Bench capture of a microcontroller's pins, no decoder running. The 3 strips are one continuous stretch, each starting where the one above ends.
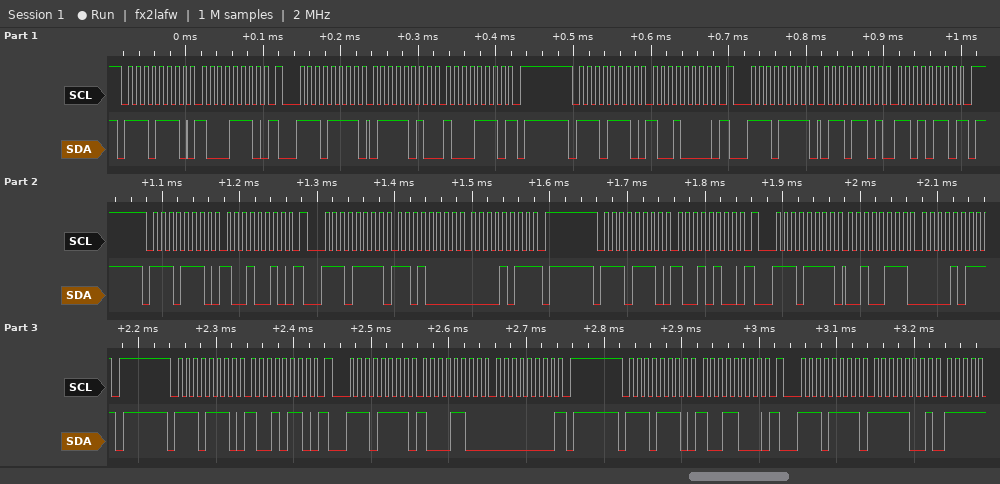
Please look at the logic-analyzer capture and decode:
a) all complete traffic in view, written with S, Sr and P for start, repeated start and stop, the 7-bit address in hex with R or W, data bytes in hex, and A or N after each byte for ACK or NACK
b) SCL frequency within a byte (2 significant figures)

S 77W A 8E A Sr 77R A 7A A 8E N P S 77W A 90 A Sr 77R A 6D A D6 N P S 77W A 92 A Sr 77R A D0 A 0B N P S 77W A 94 A Sr 77R A 27 A 0B N P S 77W A 96 A Sr 77R A 8C A 00 N P S 77W A 98 A Sr 77R A F9 A
100 kHz
